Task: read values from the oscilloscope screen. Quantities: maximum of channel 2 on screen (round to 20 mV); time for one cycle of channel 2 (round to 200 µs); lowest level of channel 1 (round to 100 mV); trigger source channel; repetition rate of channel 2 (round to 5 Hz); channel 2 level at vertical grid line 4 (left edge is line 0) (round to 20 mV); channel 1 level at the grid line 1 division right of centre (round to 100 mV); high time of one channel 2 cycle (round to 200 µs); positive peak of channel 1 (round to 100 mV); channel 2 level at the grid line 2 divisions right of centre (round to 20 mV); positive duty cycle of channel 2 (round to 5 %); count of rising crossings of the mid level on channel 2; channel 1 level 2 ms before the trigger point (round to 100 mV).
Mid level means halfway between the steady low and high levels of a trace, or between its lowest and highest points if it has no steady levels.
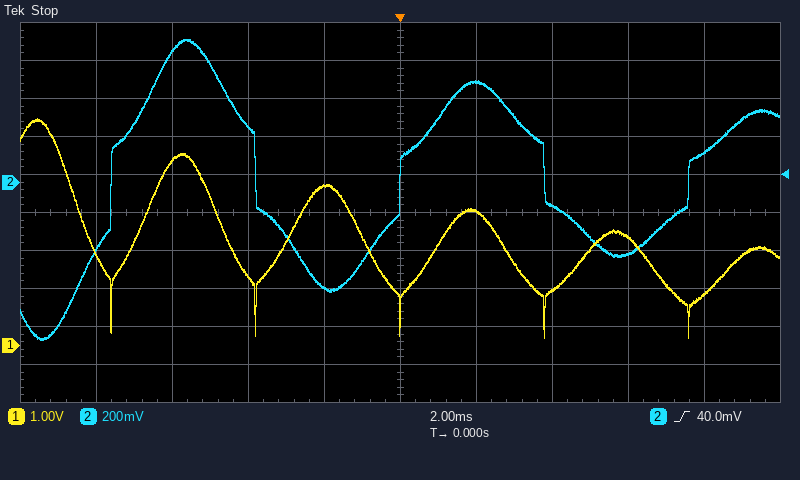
760 mV
7.6 ms
200 mV
channel 2
130 Hz
-560 mV
3.5 V
3.8 ms
6.0 V
-120 mV
50 %
3
4.2 V
